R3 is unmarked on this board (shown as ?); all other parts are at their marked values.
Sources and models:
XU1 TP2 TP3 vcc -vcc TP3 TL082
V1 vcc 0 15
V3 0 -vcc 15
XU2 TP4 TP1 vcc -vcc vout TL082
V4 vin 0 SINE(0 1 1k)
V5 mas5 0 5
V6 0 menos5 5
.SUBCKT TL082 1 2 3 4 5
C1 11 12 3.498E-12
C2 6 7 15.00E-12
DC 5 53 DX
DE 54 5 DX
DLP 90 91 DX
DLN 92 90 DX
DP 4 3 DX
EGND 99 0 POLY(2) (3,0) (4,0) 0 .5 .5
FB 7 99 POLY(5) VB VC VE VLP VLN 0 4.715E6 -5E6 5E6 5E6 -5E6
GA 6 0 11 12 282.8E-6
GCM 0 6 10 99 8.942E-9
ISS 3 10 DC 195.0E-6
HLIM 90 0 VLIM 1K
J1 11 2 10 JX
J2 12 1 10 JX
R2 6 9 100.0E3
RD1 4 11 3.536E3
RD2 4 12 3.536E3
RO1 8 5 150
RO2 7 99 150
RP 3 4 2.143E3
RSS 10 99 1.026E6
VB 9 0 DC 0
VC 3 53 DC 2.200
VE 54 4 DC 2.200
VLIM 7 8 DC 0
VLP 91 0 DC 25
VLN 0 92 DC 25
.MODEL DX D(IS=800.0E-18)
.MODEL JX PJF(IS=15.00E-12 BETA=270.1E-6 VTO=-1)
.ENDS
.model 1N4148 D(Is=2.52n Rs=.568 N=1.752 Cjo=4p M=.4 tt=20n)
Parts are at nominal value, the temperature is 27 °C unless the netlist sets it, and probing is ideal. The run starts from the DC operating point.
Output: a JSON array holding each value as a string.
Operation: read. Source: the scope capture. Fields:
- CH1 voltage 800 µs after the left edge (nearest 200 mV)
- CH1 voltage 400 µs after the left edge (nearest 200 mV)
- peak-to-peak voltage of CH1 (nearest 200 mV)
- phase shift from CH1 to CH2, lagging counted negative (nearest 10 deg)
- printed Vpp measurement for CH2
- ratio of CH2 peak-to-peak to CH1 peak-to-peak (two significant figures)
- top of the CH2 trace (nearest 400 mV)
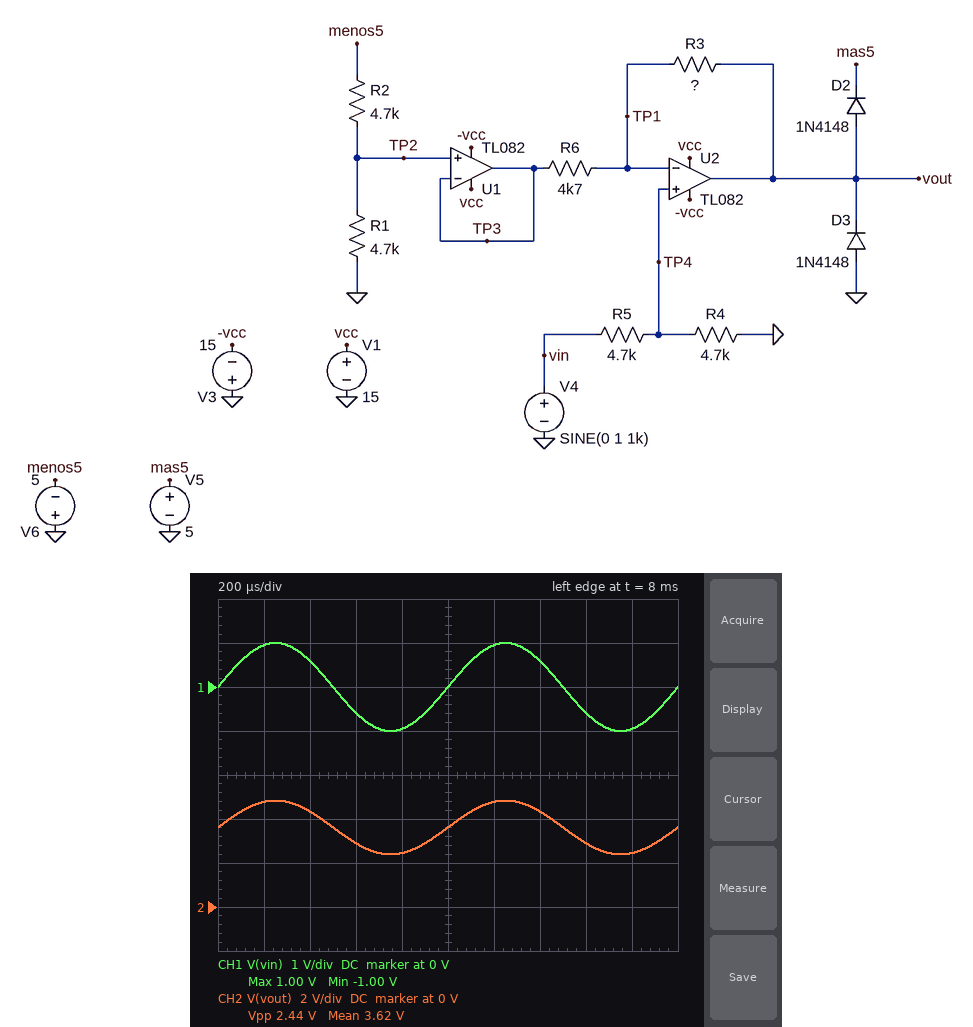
["-1.0 V", "600 mV", "2.0 V", "0 deg", "2.44 V", "1.2", "4.8 V"]
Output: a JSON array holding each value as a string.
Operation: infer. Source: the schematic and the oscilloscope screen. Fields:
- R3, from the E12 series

["6.8 kΩ"]
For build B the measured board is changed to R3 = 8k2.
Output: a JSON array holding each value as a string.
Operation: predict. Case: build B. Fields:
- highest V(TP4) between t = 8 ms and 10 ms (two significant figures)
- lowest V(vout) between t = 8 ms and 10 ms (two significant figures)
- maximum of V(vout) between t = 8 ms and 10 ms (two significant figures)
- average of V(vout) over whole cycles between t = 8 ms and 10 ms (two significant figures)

["500 mV", "3.0 V", "5.7 V", "4.4 V"]
